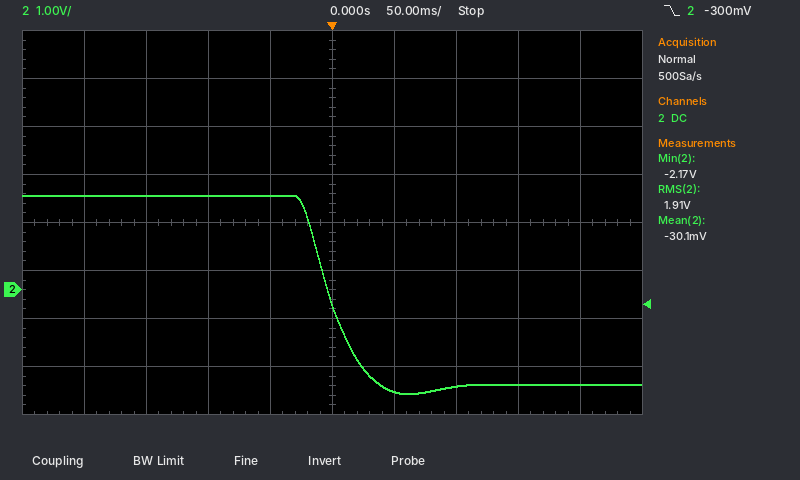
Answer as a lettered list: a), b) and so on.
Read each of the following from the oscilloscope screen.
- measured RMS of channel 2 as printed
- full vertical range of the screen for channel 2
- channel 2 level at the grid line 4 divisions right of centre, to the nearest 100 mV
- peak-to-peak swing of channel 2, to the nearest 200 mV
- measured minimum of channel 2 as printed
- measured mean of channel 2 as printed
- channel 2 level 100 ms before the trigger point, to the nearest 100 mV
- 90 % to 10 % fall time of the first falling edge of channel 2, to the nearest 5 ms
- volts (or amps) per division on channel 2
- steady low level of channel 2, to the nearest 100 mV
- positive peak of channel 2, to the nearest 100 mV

a) 1.91 V
b) 8 V
c) -2.0 V
d) 4.2 V
e) -2.17 V
f) -30.1 mV
g) 2.0 V
h) 45 ms
i) 1 V
j) -2.0 V
k) 2.0 V
